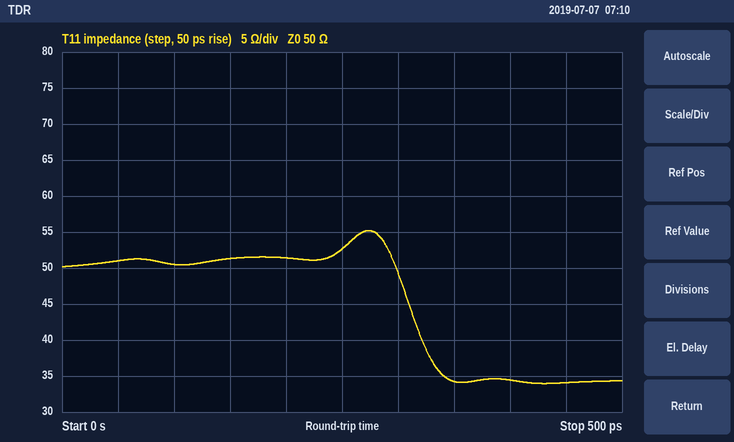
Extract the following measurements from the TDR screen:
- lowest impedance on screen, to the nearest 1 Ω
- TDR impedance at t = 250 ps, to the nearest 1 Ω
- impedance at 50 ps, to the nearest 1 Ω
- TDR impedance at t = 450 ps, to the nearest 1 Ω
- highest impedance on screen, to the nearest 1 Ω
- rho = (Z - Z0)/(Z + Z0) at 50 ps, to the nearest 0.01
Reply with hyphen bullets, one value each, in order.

- 34 Ω
- 53 Ω
- 51 Ω
- 34 Ω
- 55 Ω
- +0.01
